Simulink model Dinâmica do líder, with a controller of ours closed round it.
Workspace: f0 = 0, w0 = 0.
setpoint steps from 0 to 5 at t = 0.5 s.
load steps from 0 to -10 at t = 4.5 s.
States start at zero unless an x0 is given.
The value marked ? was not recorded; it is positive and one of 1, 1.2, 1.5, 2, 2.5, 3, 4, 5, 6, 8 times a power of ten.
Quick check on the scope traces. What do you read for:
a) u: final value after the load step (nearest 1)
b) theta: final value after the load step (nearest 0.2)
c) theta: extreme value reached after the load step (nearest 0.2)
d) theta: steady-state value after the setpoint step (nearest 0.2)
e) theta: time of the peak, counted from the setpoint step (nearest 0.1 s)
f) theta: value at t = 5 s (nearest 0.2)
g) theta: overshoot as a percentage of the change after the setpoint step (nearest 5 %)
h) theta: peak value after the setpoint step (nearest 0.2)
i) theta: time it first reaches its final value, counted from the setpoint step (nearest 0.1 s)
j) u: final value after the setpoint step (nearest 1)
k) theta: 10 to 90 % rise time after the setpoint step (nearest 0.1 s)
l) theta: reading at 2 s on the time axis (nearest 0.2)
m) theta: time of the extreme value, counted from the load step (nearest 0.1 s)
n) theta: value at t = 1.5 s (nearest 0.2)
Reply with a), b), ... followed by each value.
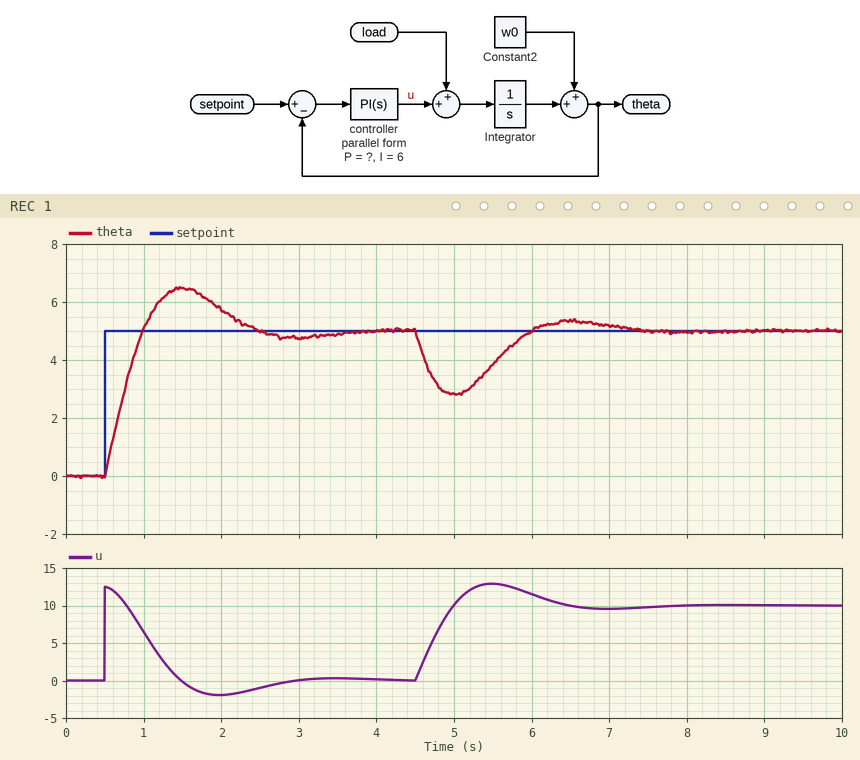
a) 10
b) 5.0
c) 2.8
d) 5.0
e) 1.0 s
f) 2.8
g) 30 %
h) 6.4
i) 0.5 s
j) 0
k) 0.4 s
l) 5.8
m) 0.5 s
n) 6.4
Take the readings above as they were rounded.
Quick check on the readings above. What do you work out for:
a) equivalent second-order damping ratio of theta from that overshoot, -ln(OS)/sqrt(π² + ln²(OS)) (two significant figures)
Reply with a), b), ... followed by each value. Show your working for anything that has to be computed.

a) ln(0.3) = -1.204; 1.204 / sqrt(9.870 + 1.450) = 0.36
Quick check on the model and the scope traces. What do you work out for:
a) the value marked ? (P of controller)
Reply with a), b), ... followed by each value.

a) 2.5
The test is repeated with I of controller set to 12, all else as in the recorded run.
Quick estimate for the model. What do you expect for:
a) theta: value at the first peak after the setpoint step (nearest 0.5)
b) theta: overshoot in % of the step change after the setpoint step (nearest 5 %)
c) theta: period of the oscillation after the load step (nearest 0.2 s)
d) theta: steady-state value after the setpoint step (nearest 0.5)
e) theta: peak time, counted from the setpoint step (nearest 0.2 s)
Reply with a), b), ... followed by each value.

a) 7.0
b) 40 %
c) 2.0 s
d) 5.0
e) 0.8 s
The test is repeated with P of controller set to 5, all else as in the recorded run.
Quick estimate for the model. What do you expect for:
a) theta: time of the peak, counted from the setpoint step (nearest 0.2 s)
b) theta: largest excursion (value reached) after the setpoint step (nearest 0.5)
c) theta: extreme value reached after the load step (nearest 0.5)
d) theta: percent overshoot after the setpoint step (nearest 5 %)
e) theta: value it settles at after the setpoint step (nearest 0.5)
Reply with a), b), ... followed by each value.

a) 0.8 s
b) 5.5
c) 3.5
d) 15 %
e) 5.0
